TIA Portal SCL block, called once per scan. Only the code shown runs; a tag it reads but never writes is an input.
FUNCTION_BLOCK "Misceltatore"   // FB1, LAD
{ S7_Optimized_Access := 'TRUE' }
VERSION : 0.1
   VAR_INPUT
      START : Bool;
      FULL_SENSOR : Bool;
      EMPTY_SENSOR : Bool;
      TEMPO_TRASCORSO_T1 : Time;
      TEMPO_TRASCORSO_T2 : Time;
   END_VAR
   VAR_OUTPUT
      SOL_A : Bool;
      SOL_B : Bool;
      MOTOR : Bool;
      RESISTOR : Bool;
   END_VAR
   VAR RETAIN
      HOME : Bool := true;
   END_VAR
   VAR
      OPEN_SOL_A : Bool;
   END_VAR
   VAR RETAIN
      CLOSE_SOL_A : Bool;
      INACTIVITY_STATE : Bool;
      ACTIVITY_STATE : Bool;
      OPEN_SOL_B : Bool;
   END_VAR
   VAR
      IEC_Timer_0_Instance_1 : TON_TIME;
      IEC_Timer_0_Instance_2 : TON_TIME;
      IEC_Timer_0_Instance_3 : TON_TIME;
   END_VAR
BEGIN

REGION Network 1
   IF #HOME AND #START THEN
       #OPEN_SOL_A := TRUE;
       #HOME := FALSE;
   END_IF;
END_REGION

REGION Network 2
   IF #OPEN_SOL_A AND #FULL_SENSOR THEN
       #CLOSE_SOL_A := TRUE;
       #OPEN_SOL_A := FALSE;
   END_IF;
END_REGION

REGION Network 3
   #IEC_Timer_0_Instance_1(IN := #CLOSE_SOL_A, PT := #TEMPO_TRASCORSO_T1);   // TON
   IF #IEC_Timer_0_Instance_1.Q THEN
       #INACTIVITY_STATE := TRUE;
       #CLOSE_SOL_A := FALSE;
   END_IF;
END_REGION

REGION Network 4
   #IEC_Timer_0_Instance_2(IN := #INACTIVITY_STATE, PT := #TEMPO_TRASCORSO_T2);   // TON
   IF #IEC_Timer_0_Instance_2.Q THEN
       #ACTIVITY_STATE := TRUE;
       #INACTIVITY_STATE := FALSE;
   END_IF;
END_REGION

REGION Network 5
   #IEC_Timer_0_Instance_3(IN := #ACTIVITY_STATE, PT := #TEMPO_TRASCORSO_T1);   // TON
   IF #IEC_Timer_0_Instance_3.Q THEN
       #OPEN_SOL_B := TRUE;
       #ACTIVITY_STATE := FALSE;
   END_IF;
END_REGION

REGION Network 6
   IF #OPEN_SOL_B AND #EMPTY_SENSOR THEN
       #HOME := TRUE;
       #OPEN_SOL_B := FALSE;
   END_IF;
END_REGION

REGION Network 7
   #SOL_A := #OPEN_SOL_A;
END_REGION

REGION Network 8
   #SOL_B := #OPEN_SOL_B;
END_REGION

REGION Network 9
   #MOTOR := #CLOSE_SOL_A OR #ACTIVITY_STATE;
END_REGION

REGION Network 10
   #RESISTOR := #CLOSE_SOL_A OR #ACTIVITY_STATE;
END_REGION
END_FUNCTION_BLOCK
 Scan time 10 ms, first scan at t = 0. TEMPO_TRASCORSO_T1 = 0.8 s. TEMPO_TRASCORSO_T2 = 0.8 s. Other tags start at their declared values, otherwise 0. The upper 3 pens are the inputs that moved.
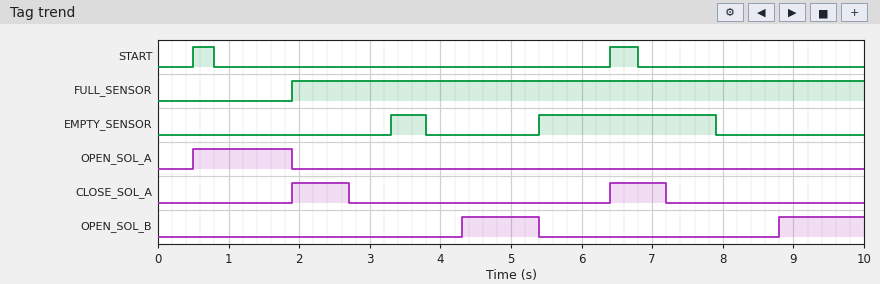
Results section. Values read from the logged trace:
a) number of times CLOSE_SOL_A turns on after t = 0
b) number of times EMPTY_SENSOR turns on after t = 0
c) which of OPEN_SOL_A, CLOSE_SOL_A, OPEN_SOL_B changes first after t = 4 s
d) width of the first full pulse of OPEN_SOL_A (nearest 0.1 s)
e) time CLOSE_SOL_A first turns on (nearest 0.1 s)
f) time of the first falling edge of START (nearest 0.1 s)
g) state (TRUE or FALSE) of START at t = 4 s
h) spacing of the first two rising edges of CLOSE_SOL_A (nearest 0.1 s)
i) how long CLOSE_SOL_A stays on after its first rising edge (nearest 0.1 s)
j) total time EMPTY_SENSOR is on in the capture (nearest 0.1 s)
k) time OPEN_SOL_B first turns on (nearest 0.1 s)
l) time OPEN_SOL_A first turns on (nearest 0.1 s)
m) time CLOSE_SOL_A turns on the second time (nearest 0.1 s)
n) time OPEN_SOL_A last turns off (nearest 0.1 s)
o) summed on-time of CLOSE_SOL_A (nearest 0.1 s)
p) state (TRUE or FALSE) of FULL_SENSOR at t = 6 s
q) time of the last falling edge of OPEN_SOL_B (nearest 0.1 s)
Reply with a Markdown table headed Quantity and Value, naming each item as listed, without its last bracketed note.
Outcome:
| Quantity | Value |
|---|---|
| number of times CLOSE_SOL_A turns on after t = 0 | 2 |
| number of times EMPTY_SENSOR turns on after t = 0 | 2 |
| which of OPEN_SOL_A, CLOSE_SOL_A, OPEN_SOL_B changes first after t = 4 s | OPEN_SOL_B |
| width of the first full pulse of OPEN_SOL_A | 1.4 s |
| time CLOSE_SOL_A first turns on | 1.9 s |
| time of the first falling edge of START | 0.8 s |
| state (TRUE or FALSE) of START at t = 4 s | FALSE |
| spacing of the first two rising edges of CLOSE_SOL_A | 4.5 s |
| how long CLOSE_SOL_A stays on after its first rising edge | 0.8 s |
| total time EMPTY_SENSOR is on in the capture | 3.0 s |
| time OPEN_SOL_B first turns on | 4.3 s |
| time OPEN_SOL_A first turns on | 0.5 s |
| time CLOSE_SOL_A turns on the second time | 6.4 s |
| time OPEN_SOL_A last turns off | 1.9 s |
| summed on-time of CLOSE_SOL_A | 1.6 s |
| state (TRUE or FALSE) of FULL_SENSOR at t = 6 s | TRUE |
| time of the last falling edge of OPEN_SOL_B | 5.4 s |
